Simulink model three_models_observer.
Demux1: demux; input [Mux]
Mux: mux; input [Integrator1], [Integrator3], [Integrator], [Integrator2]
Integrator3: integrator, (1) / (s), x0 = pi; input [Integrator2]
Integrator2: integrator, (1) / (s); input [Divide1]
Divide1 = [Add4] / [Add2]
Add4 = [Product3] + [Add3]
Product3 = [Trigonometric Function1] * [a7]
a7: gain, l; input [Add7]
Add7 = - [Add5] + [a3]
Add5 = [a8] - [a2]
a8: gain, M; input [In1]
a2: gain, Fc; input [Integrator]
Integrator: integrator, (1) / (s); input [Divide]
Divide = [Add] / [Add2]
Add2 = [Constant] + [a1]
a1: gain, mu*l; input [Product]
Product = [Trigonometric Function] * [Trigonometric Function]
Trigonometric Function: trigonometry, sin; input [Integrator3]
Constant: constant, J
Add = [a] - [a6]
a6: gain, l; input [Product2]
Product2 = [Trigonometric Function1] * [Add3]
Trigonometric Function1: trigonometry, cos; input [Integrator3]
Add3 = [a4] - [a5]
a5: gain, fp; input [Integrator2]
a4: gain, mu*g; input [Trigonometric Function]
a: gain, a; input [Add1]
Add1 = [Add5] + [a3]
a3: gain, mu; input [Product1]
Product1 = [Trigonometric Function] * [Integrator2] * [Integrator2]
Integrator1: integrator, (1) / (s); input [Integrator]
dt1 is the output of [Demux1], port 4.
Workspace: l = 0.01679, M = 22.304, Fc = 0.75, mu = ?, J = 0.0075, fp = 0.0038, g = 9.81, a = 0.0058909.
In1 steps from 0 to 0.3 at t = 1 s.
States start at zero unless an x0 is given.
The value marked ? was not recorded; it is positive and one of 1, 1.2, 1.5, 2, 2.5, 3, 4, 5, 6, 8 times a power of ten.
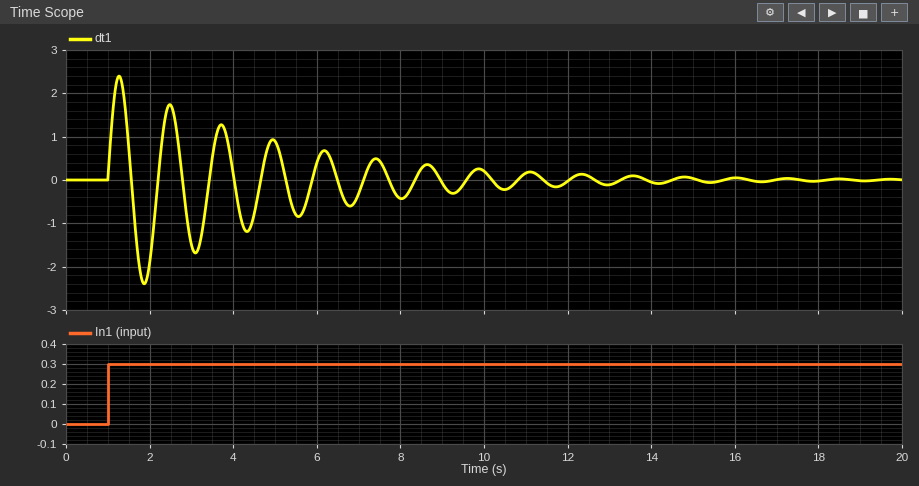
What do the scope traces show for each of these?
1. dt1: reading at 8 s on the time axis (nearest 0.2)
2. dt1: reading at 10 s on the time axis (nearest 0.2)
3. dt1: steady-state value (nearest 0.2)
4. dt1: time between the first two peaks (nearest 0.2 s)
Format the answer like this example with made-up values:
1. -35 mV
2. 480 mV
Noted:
1. -0.4
2. 0.2
3. 0.0
4. 1.2 s
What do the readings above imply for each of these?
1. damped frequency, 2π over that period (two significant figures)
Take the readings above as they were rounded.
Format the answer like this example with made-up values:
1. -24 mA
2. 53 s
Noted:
1. 5.2 rad/s
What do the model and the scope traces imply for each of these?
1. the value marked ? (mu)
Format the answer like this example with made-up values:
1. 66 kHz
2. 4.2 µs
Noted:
1. 0.02
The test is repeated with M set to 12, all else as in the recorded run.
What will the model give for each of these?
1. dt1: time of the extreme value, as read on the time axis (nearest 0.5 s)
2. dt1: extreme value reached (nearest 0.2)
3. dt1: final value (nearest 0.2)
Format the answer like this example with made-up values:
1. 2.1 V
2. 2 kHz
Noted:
1. 2.0 s
2. -1.4
3. 0.0
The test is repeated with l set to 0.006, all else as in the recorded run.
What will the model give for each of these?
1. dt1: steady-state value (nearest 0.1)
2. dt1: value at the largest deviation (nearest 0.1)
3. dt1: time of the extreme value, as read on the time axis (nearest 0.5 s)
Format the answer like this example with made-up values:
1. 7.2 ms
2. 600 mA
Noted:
1. 0.0
2. -0.9
3. 2.0 s
